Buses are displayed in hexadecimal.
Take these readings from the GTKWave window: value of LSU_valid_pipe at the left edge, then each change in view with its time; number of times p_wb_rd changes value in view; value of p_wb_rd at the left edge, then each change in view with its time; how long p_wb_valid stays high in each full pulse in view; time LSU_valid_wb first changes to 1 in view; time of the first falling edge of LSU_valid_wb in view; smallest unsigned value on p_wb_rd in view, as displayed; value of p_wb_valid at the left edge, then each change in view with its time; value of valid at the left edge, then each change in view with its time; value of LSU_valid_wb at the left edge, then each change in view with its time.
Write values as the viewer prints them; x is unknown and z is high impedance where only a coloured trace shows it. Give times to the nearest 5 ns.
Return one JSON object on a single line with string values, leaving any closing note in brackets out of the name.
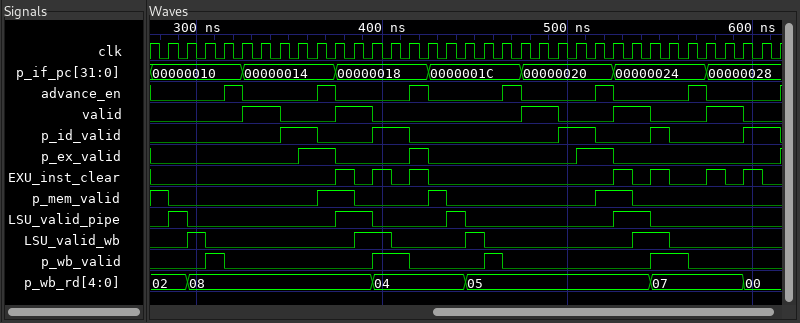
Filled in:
{"value of LSU_valid_pipe at the left edge, then each change in view with its time": "0, 1 at 285 ns, 0 at 295 ns, 1 at 375 ns, 0 at 395 ns, 1 at 435 ns, 0 at 445 ns, 1 at 525 ns, 0 at 545 ns", "number of times p_wb_rd changes value in view": "5", "value of p_wb_rd at the left edge, then each change in view with its time": "02, 08 at 295 ns, 04 at 395 ns, 05 at 445 ns, 07 at 545 ns, 00 at 595 ns", "how long p_wb_valid stays high in each full pulse in view": "10 ns, 20 ns, 10 ns, 20 ns", "time LSU_valid_wb first changes to 1 in view": "295 ns", "time of the first falling edge of LSU_valid_wb in view": "305 ns", "smallest unsigned value on p_wb_rd in view, as displayed": "00", "value of p_wb_valid at the left edge, then each change in view with its time": "0, 1 at 305 ns, 0 at 315 ns, 1 at 395 ns, 0 at 415 ns, 1 at 455 ns, 0 at 465 ns, 1 at 545 ns, 0 at 565 ns", "value of valid at the left edge, then each change in view with its time": "0, 1 at 325 ns, 0 at 345 ns, 1 at 375 ns, 0 at 395 ns, 1 at 475 ns, 0 at 495 ns, 1 at 525 ns, 0 at 545 ns, 1 at 575 ns, 0 at 595 ns", "value of LSU_valid_wb at the left edge, then each change in view with its time": "0, 1 at 295 ns, 0 at 305 ns, 1 at 385 ns, 0 at 405 ns, 1 at 445 ns, 0 at 455 ns, 1 at 535 ns, 0 at 555 ns"}
